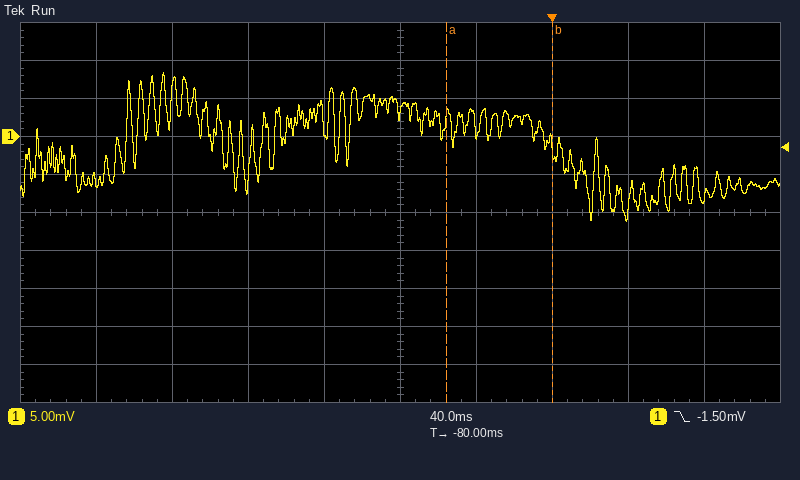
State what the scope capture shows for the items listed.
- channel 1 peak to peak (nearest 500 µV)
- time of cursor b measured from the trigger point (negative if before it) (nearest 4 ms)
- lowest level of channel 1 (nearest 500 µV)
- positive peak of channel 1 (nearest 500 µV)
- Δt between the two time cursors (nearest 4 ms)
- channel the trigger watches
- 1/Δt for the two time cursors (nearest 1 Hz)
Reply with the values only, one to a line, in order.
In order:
19.5 mV
0 ms
-11.0 mV
8.5 mV
56 ms
channel 1
18 Hz
